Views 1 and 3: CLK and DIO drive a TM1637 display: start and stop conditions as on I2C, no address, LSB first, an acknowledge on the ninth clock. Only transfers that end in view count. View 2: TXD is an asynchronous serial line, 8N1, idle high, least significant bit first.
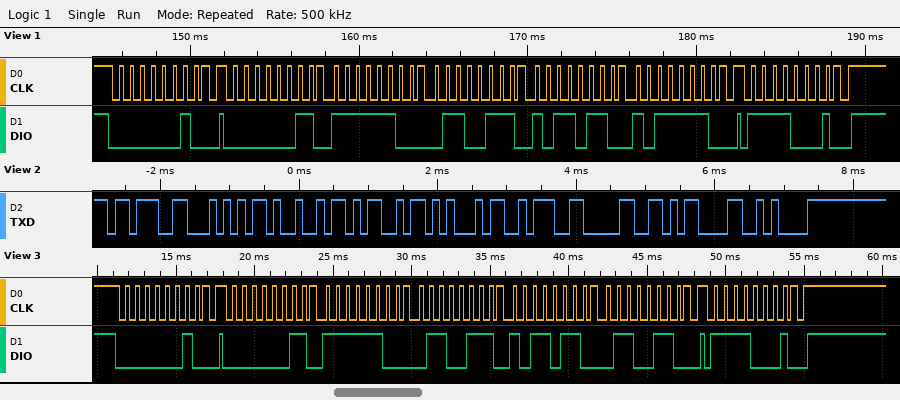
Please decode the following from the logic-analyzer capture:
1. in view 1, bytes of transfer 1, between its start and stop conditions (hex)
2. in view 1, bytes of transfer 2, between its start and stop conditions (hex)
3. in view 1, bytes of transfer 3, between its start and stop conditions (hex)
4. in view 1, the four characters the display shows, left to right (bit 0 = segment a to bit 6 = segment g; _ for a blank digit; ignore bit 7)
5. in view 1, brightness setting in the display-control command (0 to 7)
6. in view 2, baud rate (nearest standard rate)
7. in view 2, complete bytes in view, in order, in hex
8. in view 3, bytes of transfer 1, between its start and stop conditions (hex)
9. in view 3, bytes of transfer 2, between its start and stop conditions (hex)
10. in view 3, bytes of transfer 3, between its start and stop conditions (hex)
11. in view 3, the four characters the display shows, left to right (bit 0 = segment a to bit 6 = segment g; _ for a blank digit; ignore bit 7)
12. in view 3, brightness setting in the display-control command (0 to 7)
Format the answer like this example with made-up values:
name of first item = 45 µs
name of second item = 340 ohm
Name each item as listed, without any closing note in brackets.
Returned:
in view 1, bytes of transfer 1, between its start and stop conditions = 40
in view 1, bytes of transfer 2, between its start and stop conditions = C0 3F E6 6D 7D
in view 1, bytes of transfer 3, between its start and stop conditions = 8F
in view 1, the four characters the display shows, left to right = 0456
in view 1, brightness setting in the display-control command = 7
in view 2, baud rate = 9600 baud
in view 2, complete bytes in view, in order, in hex = 0x3B 0x54 0x49 0x4D 0x45 0x3A 0x30 0x0D 0x0A
in view 3, bytes of transfer 1, between its start and stop conditions = 40
in view 3, bytes of transfer 2, between its start and stop conditions = C0 3F E6 6D 66
in view 3, bytes of transfer 3, between its start and stop conditions = 8F
in view 3, the four characters the display shows, left to right = 0454
in view 3, brightness setting in the display-control command = 7
